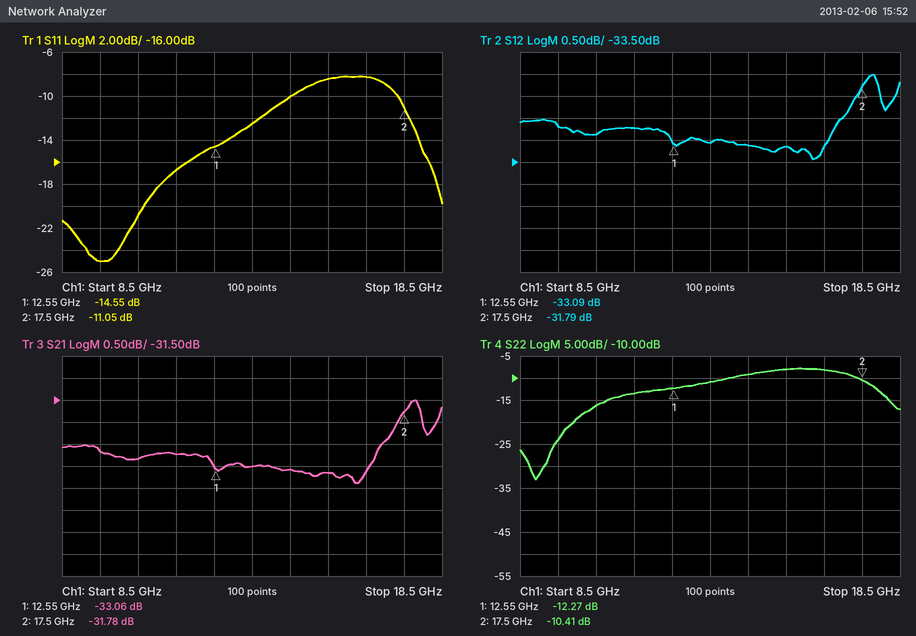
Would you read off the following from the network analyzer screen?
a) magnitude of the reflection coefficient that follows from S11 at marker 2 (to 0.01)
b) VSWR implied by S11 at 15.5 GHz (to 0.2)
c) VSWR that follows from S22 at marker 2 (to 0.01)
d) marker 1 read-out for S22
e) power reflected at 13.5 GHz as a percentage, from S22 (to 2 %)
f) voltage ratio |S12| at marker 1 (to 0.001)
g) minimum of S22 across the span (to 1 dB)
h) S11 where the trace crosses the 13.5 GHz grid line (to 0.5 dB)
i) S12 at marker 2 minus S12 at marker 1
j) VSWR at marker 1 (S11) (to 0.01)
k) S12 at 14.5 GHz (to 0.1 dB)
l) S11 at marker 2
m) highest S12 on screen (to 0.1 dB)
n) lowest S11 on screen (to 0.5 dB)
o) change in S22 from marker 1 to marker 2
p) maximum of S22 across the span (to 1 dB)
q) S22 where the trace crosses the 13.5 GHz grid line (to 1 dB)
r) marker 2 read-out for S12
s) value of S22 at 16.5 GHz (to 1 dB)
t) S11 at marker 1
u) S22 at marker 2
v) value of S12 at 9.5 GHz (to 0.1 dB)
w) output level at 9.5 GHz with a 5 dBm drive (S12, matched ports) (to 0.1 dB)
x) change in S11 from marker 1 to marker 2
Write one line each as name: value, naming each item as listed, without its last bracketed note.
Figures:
magnitude of the reflection coefficient that follows from S11 at marker 2: 0.28
VSWR implied by S11 at 15.5 GHz: 2.2
VSWR that follows from S22 at marker 2: 1.86
marker 1 read-out for S22: -12.27 dB
power reflected at 13.5 GHz as a percentage, from S22: 8 %
voltage ratio |S12| at marker 1: 0.022
minimum of S22 across the span: -33 dB
S11 where the trace crosses the 13.5 GHz grid line: -12.5 dB
S12 at marker 2 minus S12 at marker 1: 1.30 dB
VSWR at marker 1 (S11): 1.46
S12 at 14.5 GHz: -33.1 dB
S11 at marker 2: -11.05 dB
highest S12 on screen: -31.5 dB
lowest S11 on screen: -25.0 dB
change in S22 from marker 1 to marker 2: 1.86 dB
maximum of S22 across the span: -8 dB
S22 where the trace crosses the 13.5 GHz grid line: -11 dB
marker 2 read-out for S12: -31.79 dB
value of S22 at 16.5 GHz: -8 dB
S11 at marker 1: -14.55 dB
S22 at marker 2: -10.41 dB
value of S12 at 9.5 GHz: -32.7 dB
output level at 9.5 GHz with a 5 dBm drive (S12, matched ports): -27.7 dBm
change in S11 from marker 1 to marker 2: 3.50 dB
